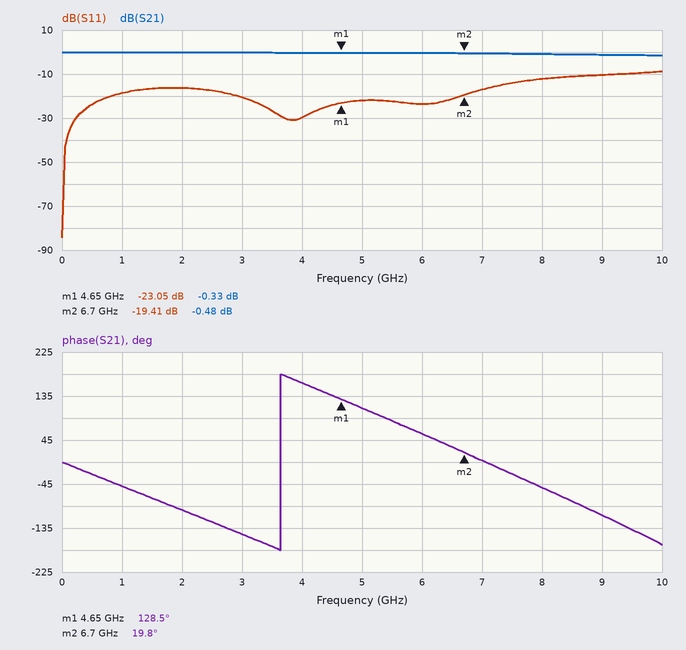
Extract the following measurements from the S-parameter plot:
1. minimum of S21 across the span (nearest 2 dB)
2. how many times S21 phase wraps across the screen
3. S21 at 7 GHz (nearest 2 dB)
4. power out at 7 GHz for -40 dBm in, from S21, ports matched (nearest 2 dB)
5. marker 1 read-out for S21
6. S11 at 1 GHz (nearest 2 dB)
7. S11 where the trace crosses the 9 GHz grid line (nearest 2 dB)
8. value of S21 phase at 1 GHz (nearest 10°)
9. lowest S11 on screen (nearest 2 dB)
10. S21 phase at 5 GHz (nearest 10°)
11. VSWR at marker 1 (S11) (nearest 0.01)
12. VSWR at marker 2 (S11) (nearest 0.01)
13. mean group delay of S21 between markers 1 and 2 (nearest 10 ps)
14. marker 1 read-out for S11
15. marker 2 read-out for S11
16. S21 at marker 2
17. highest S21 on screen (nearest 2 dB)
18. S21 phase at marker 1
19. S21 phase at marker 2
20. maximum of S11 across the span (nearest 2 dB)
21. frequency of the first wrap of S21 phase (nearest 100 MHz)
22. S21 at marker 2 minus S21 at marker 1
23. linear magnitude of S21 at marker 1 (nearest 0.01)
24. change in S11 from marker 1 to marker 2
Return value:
-2 dB
1
0 dB
-40 dBm
-0.33 dB
-18 dB
-10 dB
-50°
-84 dB
110°
1.15
1.24
150 ps
-23.05 dB
-19.41 dB
-0.48 dB
0 dB
128.5°
19.8°
-8 dB
3.6 GHz
-0.15 dB
0.96
3.64 dB
